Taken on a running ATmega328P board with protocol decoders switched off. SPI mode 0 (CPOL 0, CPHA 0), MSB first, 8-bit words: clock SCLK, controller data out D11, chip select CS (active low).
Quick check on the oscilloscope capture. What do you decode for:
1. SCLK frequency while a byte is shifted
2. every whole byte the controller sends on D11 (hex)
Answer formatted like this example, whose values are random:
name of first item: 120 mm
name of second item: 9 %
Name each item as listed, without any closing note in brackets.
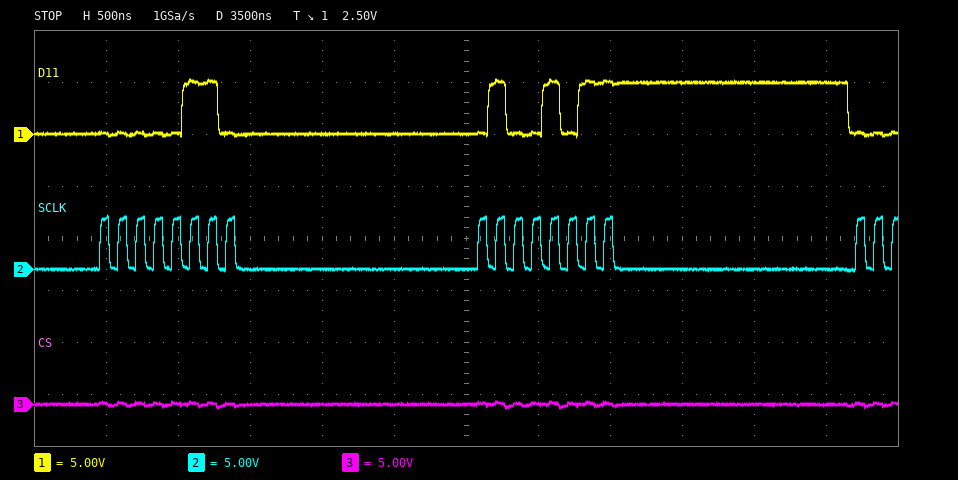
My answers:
SCLK frequency while a byte is shifted: 8 MHz
every whole byte the controller sends on D11: 06 4B
